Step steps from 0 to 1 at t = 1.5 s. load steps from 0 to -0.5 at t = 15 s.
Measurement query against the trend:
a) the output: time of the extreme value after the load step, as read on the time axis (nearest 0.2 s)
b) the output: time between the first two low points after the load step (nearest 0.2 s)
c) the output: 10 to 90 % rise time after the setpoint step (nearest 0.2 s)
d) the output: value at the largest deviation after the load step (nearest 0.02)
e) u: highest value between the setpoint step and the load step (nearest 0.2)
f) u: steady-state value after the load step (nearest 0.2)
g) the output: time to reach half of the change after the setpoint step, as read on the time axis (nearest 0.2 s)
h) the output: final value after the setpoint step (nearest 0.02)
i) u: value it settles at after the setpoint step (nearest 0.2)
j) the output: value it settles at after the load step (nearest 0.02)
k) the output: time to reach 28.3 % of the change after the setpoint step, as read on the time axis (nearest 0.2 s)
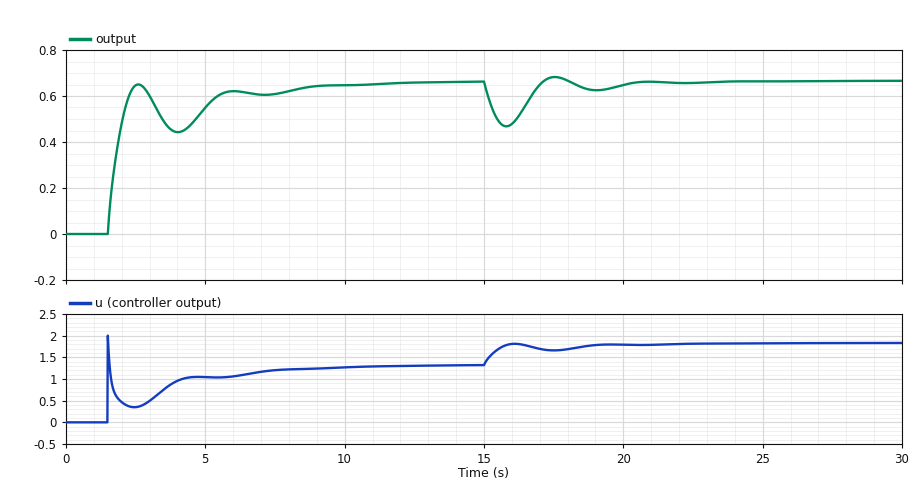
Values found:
15.8 s
3.2 s
0.8 s
0.46
2.0
1.8
1.8 s
0.66
1.4
0.66
1.6 s
